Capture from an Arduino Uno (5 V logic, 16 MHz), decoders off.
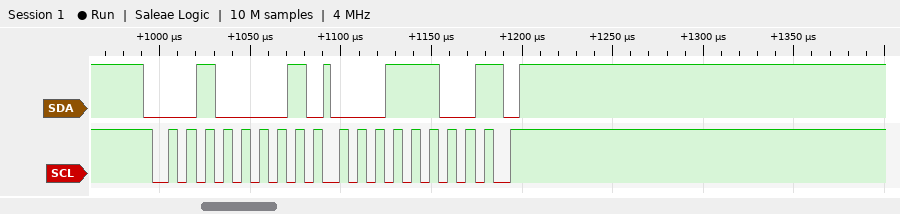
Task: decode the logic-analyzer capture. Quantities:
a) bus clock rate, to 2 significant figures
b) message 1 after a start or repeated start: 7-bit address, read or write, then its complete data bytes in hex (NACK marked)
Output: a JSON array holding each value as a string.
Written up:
["100 kHz", "0x10 read: 1C NACK"]
